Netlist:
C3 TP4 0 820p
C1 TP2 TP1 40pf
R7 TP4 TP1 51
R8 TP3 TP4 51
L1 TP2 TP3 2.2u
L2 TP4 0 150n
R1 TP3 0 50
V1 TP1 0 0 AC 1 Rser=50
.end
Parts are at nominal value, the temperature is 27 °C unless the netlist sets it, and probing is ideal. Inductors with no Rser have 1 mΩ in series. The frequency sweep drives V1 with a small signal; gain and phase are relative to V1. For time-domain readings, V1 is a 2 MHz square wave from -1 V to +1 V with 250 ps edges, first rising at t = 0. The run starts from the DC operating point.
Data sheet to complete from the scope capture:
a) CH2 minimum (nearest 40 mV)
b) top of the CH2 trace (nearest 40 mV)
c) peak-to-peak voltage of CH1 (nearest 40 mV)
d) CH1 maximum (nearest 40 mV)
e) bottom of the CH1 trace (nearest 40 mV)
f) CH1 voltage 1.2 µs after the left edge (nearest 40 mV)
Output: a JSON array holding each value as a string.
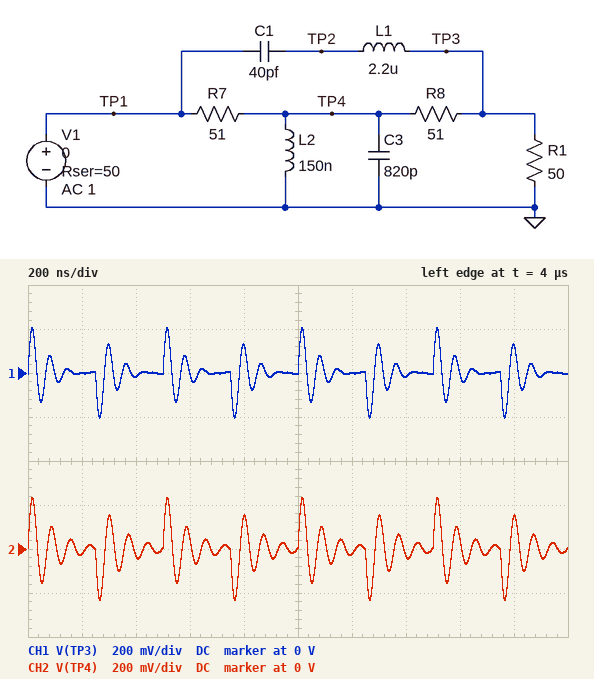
["-240 mV", "240 mV", "400 mV", "200 mV", "-200 mV", "0 V"]
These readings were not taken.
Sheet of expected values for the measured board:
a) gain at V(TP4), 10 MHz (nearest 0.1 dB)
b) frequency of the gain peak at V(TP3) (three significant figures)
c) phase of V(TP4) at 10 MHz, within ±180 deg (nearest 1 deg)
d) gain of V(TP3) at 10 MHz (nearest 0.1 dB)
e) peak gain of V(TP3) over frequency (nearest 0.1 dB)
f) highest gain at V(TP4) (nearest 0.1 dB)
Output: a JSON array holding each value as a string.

["-15.4 dB", "17.0 MHz", "70 deg", "-17.6 dB", "-8.7 dB", "-6.0 dB"]
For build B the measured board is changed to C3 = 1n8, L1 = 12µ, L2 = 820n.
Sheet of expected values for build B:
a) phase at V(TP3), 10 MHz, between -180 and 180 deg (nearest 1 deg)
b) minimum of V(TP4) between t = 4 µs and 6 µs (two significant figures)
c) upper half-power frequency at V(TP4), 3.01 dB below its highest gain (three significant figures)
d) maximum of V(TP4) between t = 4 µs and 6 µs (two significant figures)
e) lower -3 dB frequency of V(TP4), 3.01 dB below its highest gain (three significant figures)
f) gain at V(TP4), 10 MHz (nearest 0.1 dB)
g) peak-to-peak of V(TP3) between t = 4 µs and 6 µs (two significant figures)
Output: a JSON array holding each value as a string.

["-80 deg", "-250 mV", "5.11 MHz", "250 mV", "3.36 MHz", "-19.7 dB", "280 mV"]
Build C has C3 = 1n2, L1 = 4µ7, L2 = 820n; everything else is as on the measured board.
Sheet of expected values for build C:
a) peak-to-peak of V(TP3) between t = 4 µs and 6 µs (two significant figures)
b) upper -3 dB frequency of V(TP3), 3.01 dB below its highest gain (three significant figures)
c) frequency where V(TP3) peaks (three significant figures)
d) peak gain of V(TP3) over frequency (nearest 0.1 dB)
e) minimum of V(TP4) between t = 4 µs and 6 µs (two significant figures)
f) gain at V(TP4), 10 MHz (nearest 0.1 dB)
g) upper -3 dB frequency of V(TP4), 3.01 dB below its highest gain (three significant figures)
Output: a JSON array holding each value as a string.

["370 mV", "12.9 MHz", "11.8 MHz", "-11.0 dB", "-340 mV", "-15.6 dB", "6.55 MHz"]
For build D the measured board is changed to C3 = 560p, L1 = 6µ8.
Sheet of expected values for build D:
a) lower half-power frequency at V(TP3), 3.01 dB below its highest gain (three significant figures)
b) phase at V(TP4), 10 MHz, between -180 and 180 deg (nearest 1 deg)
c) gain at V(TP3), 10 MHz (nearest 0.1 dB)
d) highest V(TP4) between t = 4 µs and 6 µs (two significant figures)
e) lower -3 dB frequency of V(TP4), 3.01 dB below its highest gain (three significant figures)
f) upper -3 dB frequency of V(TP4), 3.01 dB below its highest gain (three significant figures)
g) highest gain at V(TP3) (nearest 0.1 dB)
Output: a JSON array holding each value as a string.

["8.86 MHz", "74 deg", "-13.5 dB", "260 mV", "14.8 MHz", "20.4 MHz", "-11.1 dB"]
